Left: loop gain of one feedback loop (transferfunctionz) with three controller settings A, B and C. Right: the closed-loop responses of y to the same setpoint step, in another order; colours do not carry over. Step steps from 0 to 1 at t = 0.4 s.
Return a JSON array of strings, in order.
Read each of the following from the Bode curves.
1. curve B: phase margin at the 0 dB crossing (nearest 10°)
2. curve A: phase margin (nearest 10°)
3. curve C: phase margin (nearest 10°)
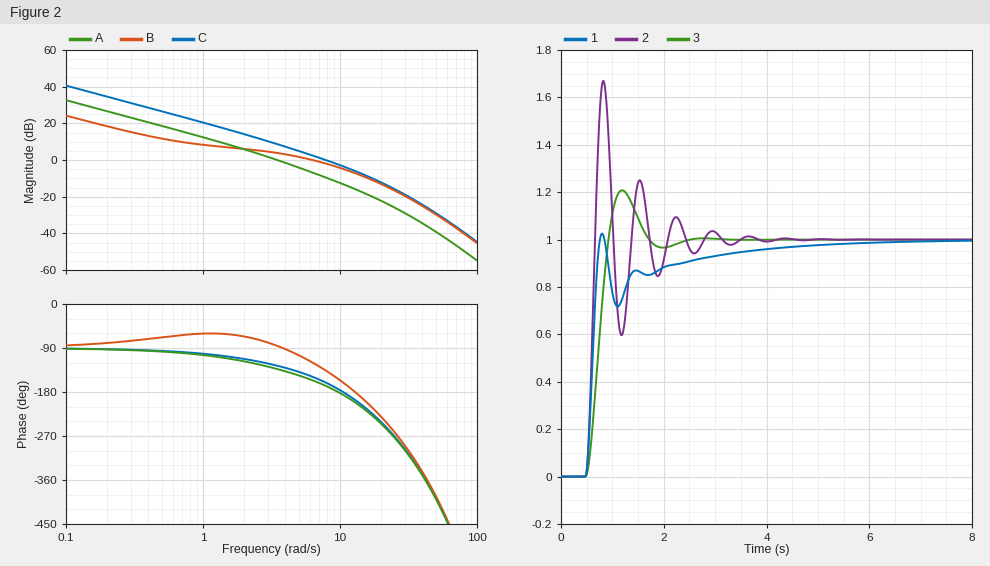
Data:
["60°", "50°", "20°"]
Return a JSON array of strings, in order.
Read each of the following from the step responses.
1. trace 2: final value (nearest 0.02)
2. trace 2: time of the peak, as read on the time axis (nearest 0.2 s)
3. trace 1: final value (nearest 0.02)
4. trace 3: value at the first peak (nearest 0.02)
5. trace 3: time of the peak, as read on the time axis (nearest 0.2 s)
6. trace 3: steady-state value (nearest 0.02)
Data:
["1.00", "0.8 s", "1.00", "1.20", "1.2 s", "1.00"]
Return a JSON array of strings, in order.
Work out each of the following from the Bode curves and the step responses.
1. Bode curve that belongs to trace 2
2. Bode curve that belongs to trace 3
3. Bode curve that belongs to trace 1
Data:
["C", "A", "B"]
